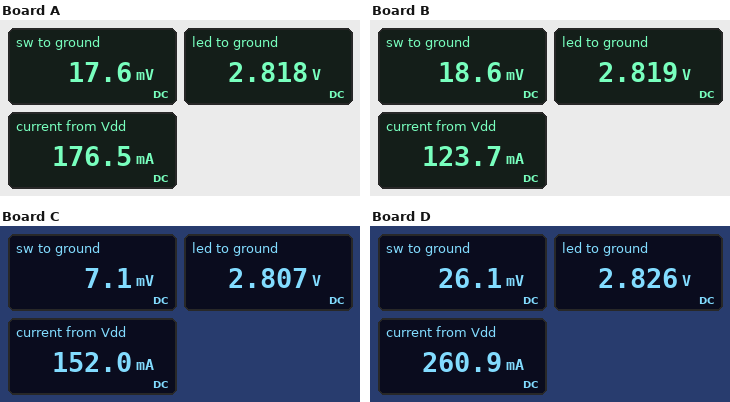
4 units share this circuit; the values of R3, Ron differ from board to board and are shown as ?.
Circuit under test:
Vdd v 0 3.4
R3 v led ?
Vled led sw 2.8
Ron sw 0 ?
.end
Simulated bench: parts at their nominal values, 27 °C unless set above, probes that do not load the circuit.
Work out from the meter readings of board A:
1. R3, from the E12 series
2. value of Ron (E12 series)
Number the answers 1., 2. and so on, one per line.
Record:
1. 3.3 Ω
2. 0.1 Ω
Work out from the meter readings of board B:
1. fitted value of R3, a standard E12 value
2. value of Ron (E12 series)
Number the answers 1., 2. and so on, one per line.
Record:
1. 4.7 Ω
2. 0.15 Ω
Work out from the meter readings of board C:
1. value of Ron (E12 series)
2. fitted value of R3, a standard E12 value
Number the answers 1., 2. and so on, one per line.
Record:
1. 0.047 Ω
2. 3.9 Ω
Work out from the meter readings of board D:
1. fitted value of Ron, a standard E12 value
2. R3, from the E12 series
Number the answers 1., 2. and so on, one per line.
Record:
1. 0.1 Ω
2. 2.2 Ω
